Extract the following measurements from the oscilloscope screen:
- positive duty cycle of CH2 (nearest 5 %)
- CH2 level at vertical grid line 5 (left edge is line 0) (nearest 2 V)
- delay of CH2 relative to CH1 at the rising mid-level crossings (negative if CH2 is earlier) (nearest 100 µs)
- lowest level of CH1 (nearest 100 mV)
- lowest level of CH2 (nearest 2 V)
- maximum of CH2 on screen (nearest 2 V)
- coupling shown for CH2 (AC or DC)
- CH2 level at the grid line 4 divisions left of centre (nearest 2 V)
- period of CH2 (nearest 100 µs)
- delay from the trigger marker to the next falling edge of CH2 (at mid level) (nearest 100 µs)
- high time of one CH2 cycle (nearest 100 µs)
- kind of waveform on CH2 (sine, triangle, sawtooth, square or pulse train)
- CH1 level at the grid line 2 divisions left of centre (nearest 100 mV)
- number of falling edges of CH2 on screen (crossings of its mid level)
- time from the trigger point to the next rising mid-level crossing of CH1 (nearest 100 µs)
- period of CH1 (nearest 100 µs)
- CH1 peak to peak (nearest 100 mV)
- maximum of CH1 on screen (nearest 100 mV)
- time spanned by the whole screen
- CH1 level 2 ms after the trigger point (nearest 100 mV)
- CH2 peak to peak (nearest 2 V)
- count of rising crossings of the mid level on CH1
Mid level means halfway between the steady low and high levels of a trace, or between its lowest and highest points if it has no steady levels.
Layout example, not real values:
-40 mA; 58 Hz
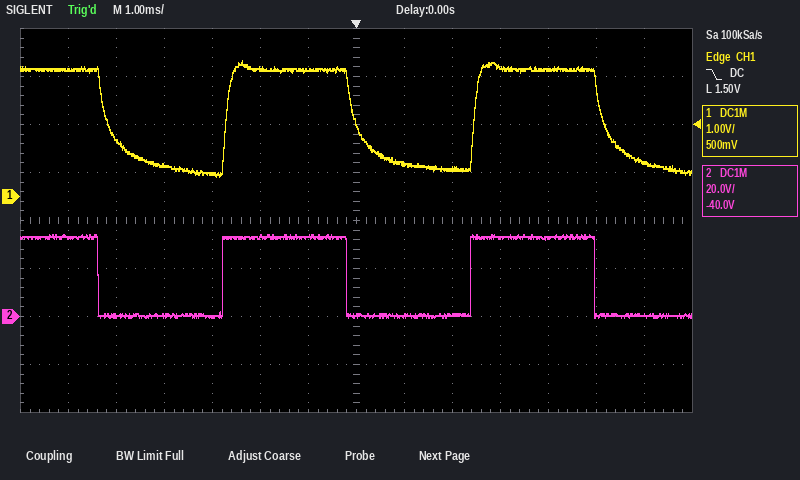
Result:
50 %; 34 V; -100 µs; 400 mV; 0 V; 34 V; DC; 0 V; 5.2 ms; 5.0 ms; 2.6 ms; square; 2.7 V; 3; 2.5 ms; 5.2 ms; 2.4 V; 2.8 V; 14 ms; 600 mV; 34 V; 2
